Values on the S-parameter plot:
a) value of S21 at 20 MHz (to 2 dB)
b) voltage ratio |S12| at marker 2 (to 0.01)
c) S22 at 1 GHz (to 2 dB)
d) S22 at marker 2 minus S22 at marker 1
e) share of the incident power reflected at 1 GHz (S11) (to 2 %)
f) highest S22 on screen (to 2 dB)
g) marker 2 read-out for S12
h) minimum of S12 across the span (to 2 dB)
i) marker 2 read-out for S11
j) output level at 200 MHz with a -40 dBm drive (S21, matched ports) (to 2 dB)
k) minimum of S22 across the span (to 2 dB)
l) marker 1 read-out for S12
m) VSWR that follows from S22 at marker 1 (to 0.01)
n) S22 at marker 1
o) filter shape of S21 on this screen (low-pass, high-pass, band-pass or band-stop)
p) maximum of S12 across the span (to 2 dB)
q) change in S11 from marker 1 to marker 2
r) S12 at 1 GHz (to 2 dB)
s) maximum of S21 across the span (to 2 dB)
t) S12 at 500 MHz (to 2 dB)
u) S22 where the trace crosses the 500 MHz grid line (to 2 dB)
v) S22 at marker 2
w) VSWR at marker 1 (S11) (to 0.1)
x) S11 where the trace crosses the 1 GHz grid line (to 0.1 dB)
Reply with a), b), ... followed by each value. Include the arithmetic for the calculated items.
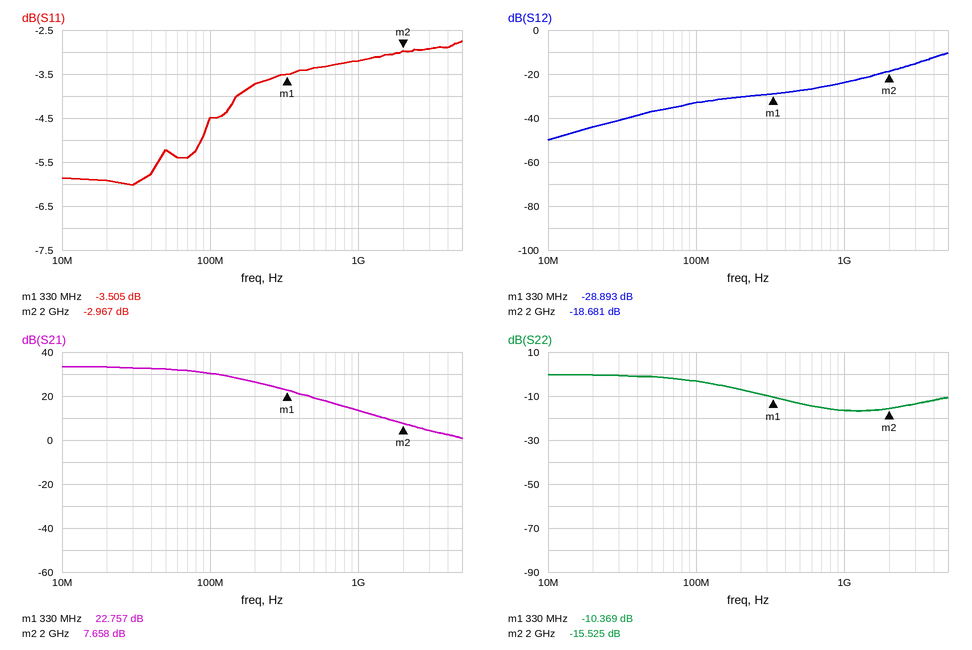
a) 34 dB
b) 10^(-18.681/20) ≈ 0.12
c) -16 dB
d) -15.525 − (-10.369) = -5.156 dB
e) 10^(-3.2/10) ≈ 48 %
f) 0 dB
g) -18.681 dB
h) -50 dB
i) -2.967 dB
j) -40 dBm + (26 dB) = -14 dBm
k) -16 dB
l) -28.893 dB
m) (1 + 0.3031)/(1 − 0.3031) ≈ 1.87
n) -10.369 dB
o) low-pass
p) -10 dB
q) -2.967 − (-3.505) = 0.538 dB
r) -24 dB
s) 34 dB
t) -28 dB
u) -14 dB
v) -15.525 dB
w) (1 + 0.6680)/(1 − 0.6680) ≈ 5.0
x) -3.2 dB
